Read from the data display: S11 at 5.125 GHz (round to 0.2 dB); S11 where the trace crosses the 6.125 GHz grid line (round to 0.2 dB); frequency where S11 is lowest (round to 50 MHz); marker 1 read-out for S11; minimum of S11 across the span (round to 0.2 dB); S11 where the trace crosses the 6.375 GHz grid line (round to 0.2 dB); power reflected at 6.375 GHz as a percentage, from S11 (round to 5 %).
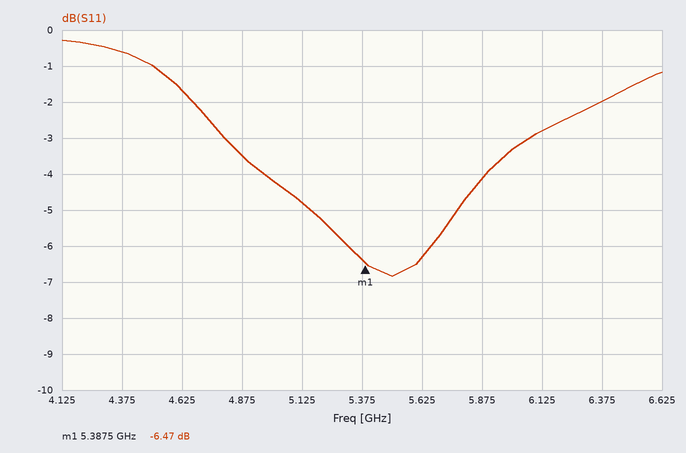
-4.8 dB
-2.8 dB
5.50 GHz
-6.47 dB
-6.8 dB
-2.0 dB
65 %
